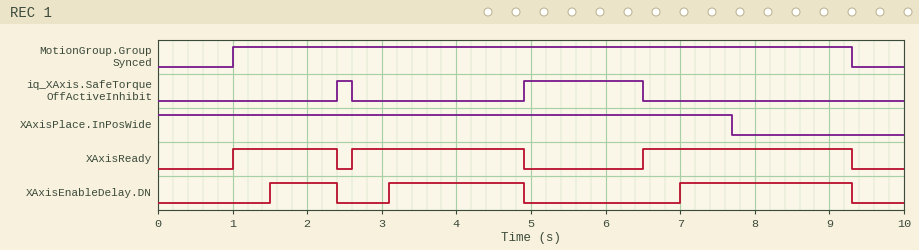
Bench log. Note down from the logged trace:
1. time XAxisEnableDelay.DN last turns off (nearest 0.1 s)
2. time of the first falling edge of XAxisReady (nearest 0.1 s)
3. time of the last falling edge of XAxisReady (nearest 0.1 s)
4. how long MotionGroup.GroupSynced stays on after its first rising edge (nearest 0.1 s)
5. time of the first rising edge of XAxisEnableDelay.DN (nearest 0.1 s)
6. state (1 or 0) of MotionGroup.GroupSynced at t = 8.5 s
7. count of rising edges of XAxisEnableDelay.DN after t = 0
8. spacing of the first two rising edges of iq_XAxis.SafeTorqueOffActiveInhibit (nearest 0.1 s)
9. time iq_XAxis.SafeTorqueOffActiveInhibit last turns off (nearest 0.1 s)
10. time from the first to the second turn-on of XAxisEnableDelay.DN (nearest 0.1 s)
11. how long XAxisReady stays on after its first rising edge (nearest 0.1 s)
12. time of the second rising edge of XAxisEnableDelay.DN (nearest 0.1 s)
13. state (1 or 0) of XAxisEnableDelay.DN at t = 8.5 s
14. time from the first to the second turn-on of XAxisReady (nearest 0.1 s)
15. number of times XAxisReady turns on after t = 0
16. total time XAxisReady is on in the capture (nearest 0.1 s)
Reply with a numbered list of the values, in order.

1. 9.3 s
2. 2.4 s
3. 9.3 s
4. 8.3 s
5. 1.5 s
6. 1
7. 3
8. 2.5 s
9. 6.5 s
10. 1.6 s
11. 1.4 s
12. 3.1 s
13. 1
14. 1.6 s
15. 3
16. 6.5 s
